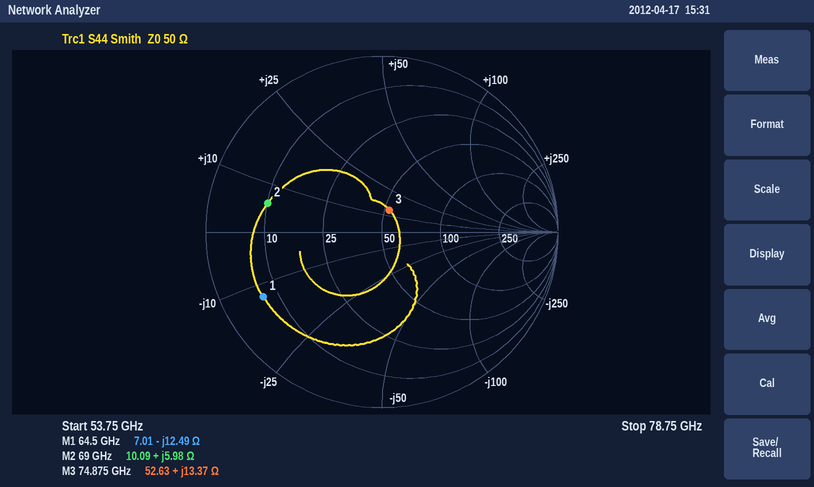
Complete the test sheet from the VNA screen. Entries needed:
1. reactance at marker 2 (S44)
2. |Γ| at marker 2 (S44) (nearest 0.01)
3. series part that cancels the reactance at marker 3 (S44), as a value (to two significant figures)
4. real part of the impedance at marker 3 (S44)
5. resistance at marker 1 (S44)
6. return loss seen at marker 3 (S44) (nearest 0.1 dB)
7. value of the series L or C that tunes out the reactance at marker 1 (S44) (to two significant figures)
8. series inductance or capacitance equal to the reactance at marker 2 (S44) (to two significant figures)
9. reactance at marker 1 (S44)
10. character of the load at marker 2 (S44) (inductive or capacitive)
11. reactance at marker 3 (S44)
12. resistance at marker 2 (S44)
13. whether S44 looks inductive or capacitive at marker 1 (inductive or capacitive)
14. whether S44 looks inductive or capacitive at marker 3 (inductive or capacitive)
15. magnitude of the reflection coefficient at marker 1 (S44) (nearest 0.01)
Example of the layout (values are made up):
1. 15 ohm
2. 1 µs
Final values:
1. +5.98 Ω
2. 0.67
3. 160 fF
4. 52.63 Ω
5. 7.01 Ω
6. 17.6 dB
7. 31 pH
8. 14 pH
9. -12.49 Ω
10. inductive
11. +13.37 Ω
12. 10.09 Ω
13. capacitive
14. inductive
15. 0.77
